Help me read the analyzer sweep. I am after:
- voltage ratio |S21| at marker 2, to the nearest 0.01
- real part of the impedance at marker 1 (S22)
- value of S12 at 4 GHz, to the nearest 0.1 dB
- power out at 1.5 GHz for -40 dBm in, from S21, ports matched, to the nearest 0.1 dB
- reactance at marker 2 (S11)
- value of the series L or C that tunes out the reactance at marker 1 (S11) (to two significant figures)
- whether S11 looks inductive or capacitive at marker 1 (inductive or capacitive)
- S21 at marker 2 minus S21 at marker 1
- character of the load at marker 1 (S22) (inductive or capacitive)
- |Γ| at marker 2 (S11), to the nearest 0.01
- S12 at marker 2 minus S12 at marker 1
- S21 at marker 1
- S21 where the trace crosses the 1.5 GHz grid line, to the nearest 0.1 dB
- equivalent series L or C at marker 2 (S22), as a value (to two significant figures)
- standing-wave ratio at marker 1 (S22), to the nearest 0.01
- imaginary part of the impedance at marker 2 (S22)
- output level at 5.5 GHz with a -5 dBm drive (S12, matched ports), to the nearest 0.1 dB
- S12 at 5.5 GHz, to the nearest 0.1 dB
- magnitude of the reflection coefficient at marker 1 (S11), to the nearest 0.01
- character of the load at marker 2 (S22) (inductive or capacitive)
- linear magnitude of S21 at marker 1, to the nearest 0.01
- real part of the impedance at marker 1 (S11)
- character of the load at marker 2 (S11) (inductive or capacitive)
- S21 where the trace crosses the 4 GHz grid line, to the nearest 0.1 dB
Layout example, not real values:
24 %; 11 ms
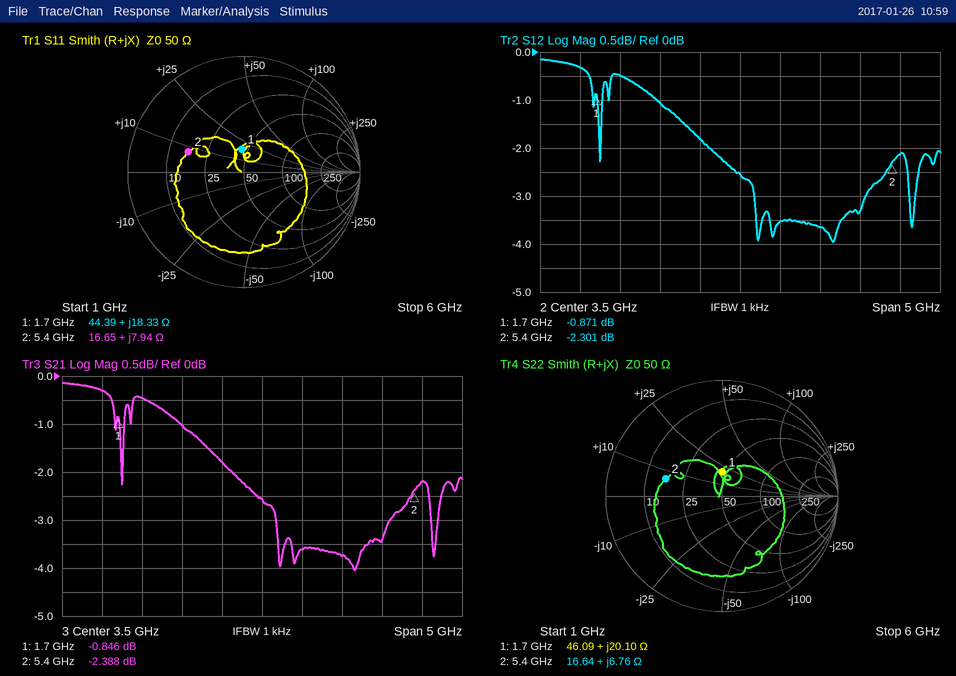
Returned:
0.76; 46.09 Ω; -3.5 dB; -40.3 dBm; +7.94 Ω; 5.1 pF; inductive; -1.542 dB; inductive; 0.51; -1.430 dB; -0.846 dB; -0.3 dB; 200 pH; 1.53; +6.76 Ω; -7.1 dBm; -2.1 dB; 0.20; inductive; 0.91; 44.39 Ω; inductive; -3.6 dB
